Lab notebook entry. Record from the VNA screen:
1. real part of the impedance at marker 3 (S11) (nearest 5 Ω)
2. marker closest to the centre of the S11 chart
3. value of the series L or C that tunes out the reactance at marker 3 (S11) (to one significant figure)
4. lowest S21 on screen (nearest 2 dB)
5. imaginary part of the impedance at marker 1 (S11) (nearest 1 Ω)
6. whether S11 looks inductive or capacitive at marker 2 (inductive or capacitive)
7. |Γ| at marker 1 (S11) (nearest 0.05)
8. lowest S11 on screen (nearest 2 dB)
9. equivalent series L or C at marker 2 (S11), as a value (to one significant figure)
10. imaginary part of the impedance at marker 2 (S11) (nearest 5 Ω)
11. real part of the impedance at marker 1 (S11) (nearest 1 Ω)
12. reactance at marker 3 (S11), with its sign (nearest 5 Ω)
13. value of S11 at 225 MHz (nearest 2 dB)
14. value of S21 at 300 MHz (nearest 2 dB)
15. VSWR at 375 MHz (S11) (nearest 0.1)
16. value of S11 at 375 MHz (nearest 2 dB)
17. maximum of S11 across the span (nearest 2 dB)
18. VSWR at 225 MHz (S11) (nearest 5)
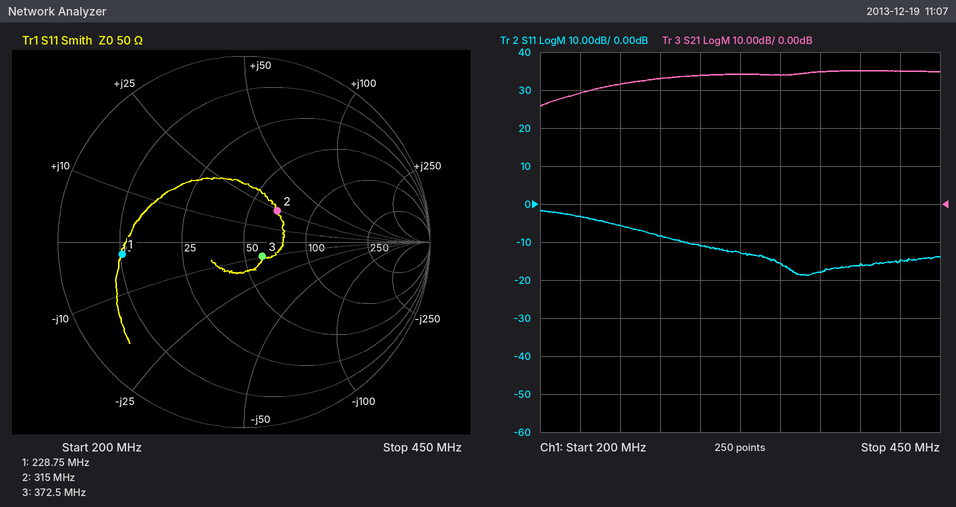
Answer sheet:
60 Ω
marker 3
4 nH
26 dB
-2 Ω
inductive
0.65
-18 dB
10 nH
+25 Ω
10 Ω
-10 Ω
-4 dB
34 dB
1.3
-18 dB
-2 dB
5
